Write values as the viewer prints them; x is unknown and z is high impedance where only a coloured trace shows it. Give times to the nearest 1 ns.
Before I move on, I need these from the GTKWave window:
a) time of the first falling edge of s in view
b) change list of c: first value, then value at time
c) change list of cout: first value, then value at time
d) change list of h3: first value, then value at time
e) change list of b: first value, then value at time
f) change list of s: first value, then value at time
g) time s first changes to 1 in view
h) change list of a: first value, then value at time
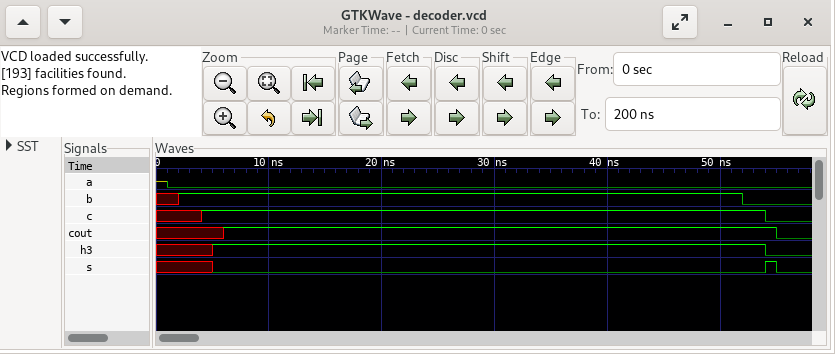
55 ns
x, 1 at 4 ns, 0 at 54 ns
x, 1 at 6 ns, 0 at 55 ns
x, 1 at 5 ns, 0 at 54 ns
x, 1 at 2 ns, 0 at 52 ns
x, 0 at 5 ns, 1 at 54 ns, 0 at 55 ns
54 ns
z, 0 at 1 ns
